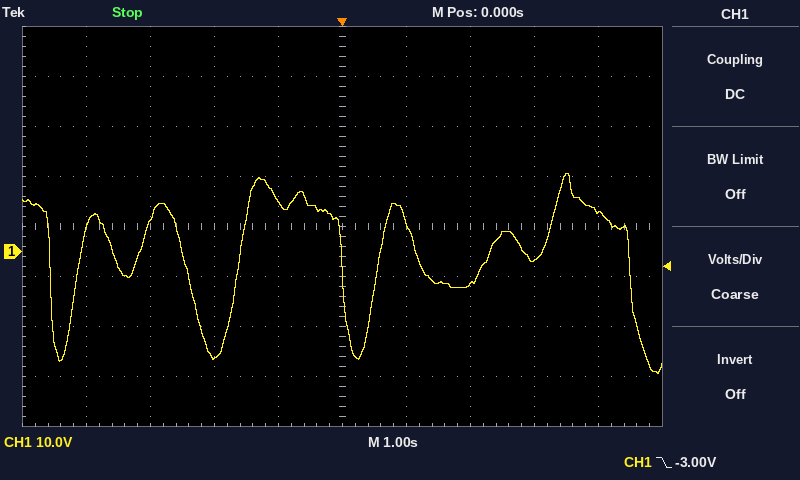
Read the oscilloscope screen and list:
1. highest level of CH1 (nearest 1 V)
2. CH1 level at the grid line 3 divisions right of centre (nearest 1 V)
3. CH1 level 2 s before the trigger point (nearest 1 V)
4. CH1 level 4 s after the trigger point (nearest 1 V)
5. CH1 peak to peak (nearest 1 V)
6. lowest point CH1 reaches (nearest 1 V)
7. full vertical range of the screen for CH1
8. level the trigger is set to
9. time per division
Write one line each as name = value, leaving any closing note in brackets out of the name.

highest level of CH1 = 16 V
CH1 level at the grid line 3 divisions right of centre = -2 V
CH1 level 2 s before the trigger point = -21 V
CH1 level 4 s after the trigger point = 8 V
CH1 peak to peak = 40 V
lowest point CH1 reaches = -24 V
full vertical range of the screen for CH1 = 80 V
level the trigger is set to = -3.00 V
time per division = 1 s
